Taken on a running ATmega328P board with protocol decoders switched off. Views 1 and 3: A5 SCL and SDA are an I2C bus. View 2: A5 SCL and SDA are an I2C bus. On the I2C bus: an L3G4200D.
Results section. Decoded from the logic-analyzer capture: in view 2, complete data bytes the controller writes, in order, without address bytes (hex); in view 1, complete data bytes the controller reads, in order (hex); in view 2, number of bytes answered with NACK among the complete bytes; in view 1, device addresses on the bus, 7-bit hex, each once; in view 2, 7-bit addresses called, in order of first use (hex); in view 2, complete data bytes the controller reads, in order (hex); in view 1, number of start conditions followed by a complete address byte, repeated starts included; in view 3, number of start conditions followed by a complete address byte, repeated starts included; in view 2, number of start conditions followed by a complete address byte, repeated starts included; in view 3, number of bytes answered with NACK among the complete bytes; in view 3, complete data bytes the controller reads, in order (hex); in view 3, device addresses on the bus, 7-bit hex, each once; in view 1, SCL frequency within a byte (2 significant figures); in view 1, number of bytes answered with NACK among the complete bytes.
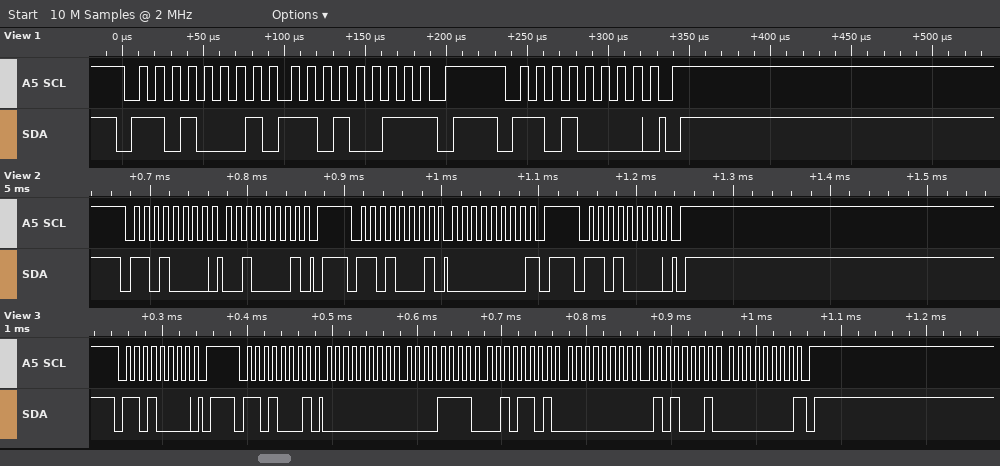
21
D3
1
0x68
0x68
00
2
2
3
1
00 0F 2D 00 51 00
0x68
100 kHz
1
